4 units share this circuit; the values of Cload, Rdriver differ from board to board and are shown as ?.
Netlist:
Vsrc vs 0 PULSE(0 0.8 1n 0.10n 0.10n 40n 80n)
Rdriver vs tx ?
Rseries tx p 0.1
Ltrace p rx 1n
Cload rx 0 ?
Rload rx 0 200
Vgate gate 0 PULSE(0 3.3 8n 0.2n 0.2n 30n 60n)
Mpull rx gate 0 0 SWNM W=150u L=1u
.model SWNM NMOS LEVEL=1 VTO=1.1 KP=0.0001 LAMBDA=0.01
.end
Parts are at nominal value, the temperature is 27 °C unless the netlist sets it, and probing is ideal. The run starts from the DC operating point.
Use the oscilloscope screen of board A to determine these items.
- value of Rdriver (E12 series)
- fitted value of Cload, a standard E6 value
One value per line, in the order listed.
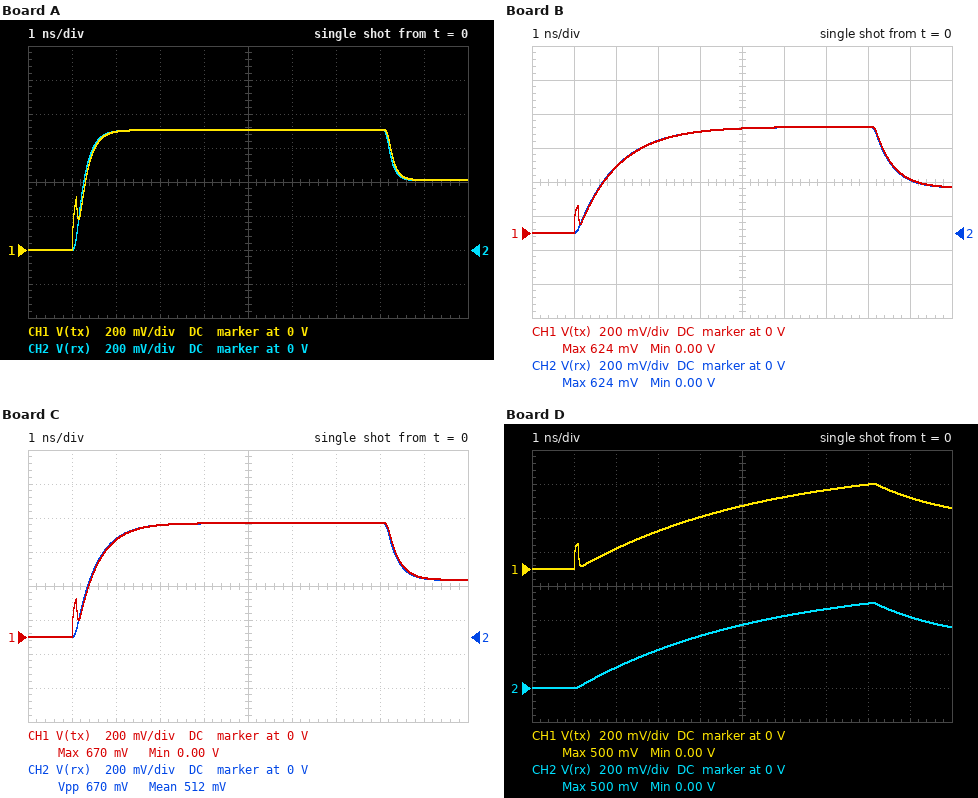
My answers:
27 Ω
10 pF
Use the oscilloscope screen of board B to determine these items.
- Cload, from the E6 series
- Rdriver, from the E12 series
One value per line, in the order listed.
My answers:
22 pF
56 Ω
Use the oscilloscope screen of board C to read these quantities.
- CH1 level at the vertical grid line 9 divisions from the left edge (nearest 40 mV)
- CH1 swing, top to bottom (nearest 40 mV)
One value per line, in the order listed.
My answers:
360 mV
680 mV
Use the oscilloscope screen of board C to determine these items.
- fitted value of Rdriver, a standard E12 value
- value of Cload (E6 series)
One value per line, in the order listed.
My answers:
39 Ω
15 pF
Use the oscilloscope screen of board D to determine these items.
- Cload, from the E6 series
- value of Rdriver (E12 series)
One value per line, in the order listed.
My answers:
100 pF
56 Ω
